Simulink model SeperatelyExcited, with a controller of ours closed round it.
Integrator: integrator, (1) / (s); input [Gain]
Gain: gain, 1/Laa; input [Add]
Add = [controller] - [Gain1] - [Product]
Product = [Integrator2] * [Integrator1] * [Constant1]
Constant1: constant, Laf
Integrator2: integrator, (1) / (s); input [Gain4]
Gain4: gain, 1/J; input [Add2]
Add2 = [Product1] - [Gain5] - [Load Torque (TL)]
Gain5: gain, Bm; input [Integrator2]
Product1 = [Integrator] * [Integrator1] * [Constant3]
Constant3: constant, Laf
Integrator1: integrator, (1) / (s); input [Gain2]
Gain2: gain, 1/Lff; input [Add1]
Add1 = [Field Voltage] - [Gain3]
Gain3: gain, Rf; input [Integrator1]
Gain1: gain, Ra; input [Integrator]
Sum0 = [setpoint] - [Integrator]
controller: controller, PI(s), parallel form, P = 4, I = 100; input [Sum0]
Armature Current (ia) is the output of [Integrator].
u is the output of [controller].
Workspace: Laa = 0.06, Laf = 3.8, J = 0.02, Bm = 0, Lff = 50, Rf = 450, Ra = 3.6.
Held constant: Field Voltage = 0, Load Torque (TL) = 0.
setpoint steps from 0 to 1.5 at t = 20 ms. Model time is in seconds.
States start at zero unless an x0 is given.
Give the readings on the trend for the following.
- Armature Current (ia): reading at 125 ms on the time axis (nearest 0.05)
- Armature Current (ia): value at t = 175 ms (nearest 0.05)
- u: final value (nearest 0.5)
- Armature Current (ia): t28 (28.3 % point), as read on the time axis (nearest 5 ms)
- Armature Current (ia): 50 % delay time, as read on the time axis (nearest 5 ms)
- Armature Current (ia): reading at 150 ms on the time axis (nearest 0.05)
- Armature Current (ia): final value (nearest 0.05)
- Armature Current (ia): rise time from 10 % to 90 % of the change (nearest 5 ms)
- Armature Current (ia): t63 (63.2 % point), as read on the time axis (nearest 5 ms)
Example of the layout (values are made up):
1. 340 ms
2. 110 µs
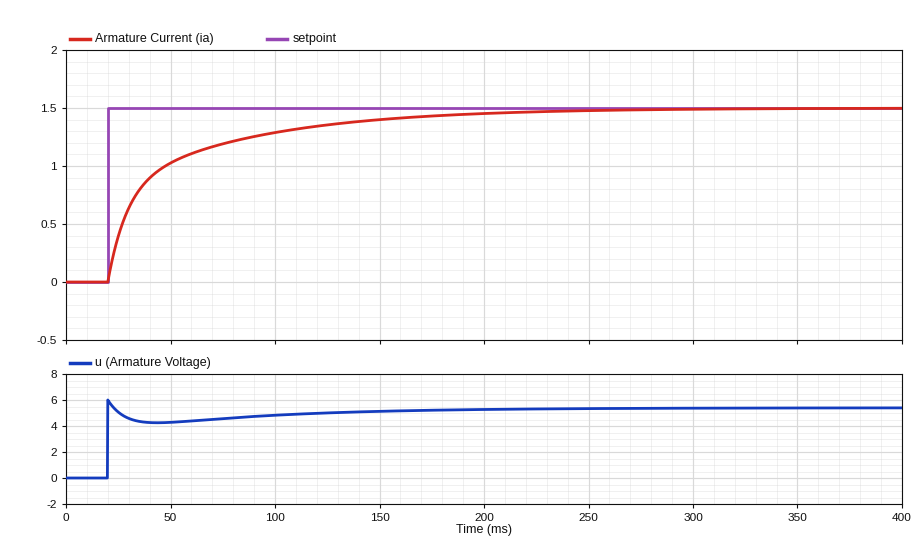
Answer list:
1. 1.35
2. 1.45
3. 5.5
4. 25 ms
5. 35 ms
6. 1.40
7. 1.50
8. 100 ms
9. 45 ms
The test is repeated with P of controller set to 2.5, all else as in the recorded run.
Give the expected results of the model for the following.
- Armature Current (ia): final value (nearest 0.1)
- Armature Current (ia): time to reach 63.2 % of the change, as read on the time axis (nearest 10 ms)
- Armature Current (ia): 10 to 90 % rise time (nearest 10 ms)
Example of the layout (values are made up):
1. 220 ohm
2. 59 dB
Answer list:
1. 1.5
2. 50 ms
3. 90 ms
